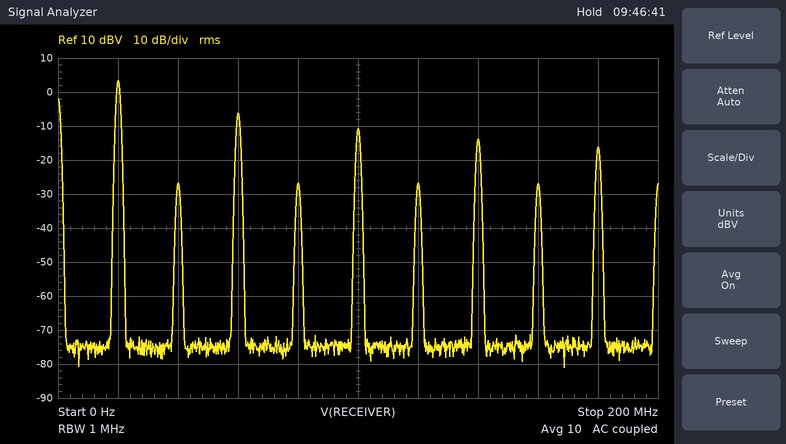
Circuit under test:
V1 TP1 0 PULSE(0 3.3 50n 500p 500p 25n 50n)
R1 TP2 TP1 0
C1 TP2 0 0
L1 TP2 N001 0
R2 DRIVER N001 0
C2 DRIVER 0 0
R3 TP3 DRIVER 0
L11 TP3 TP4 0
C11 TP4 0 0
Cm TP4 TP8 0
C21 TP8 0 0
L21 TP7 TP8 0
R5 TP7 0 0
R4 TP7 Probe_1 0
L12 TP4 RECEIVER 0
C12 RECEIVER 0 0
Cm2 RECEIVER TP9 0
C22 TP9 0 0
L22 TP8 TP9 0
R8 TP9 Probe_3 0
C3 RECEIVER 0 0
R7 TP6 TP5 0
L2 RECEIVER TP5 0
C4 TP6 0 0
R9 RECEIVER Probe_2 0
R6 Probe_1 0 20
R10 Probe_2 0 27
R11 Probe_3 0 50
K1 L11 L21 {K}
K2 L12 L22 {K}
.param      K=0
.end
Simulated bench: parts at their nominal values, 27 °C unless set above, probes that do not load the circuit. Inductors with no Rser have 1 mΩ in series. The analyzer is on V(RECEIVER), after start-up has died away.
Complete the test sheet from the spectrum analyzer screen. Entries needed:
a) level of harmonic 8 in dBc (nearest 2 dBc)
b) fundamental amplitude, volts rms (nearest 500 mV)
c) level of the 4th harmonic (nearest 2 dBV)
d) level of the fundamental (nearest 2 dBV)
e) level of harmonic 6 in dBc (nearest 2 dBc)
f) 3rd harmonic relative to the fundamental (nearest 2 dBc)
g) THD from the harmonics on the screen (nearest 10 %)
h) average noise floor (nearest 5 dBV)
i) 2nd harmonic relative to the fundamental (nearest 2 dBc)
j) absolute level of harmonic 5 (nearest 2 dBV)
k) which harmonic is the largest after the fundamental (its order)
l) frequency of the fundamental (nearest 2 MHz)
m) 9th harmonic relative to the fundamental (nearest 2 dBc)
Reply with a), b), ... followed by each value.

a) -30 dBc
b) 1.5 V
c) -26 dBV
d) 4 dBV
e) -30 dBc
f) -10 dBc
g) 40 %
h) -75 dBV
i) -30 dBc
j) -10 dBV
k) 3
l) 20 MHz
m) -20 dBc
